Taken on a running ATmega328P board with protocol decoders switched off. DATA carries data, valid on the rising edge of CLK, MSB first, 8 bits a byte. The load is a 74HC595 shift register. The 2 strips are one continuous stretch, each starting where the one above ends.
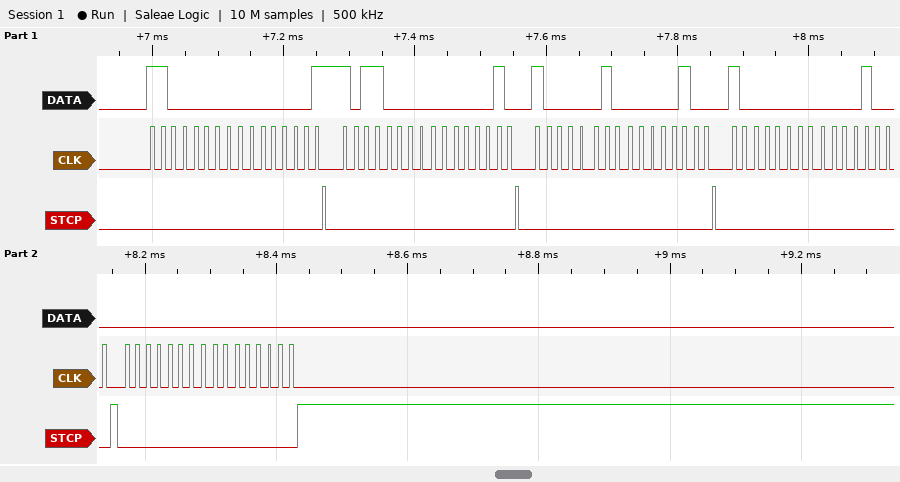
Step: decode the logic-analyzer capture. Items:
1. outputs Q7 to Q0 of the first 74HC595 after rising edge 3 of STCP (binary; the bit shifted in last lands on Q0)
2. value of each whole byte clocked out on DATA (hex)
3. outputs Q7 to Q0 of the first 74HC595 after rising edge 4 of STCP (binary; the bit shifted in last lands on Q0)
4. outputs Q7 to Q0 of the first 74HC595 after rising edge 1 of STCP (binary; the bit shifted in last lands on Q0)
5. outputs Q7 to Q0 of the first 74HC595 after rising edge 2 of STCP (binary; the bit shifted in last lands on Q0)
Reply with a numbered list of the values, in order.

1. 00000100
2. 0xC0 0x01 0xB0 0x02 0x82 0x04 0x80 0x08 0x00 0x00
3. 00001000
4. 00000001
5. 00000010
